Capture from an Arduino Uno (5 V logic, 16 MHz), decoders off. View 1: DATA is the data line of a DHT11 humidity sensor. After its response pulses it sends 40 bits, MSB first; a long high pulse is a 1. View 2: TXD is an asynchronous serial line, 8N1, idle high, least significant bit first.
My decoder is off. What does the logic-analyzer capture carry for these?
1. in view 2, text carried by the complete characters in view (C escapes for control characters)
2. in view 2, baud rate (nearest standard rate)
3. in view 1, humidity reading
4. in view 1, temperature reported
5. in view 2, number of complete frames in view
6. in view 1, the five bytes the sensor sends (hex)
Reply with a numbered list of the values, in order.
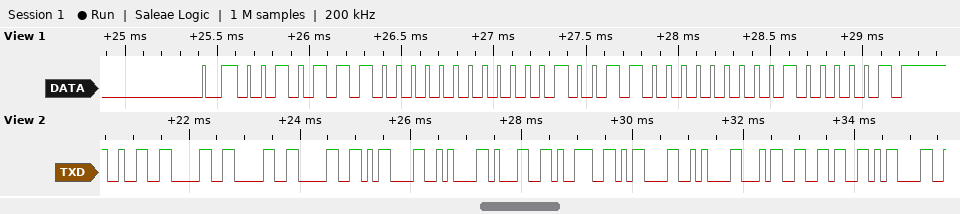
1. "2000\r\n19\r\n46\r"
2. 9600 baud
3. 46 %
4. 19.0 °C
5. 13
6. 2E 00 13 00 41
